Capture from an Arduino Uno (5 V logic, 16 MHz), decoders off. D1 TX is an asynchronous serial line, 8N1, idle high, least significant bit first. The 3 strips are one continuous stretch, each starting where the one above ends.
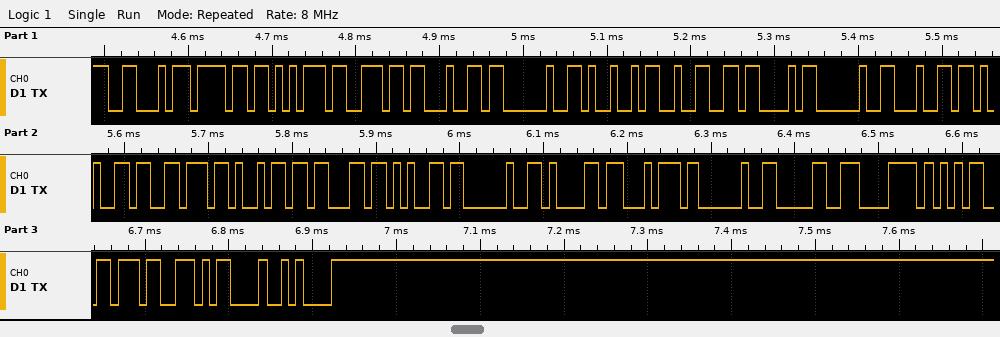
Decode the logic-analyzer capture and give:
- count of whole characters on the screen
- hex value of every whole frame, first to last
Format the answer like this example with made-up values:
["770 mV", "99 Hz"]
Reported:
["26", "46 6F 75 6E 64 20 49 32 43 20 64 65 76 69 63 65 20 61 74 20 30 78 35 37 0D 0A"]
